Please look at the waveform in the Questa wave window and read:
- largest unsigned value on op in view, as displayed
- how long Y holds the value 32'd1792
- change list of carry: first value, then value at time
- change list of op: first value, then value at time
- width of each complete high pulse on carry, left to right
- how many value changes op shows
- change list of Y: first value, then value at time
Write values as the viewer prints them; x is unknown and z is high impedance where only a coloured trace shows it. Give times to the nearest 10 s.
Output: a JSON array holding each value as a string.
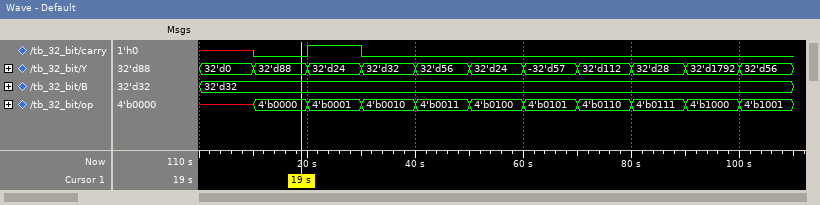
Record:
["4'b1001", "10 s", "x, 0 at 10 s, 1 at 20 s, 0 at 30 s", "x, 4'b0000 at 10 s, 4'b0001 at 20 s, 4'b0010 at 30 s, 4'b0011 at 40 s, 4'b0100 at 50 s, 4'b0101 at 60 s, 4'b0110 at 70 s, 4'b0111 at 80 s, 4'b1000 at 90 s, 4'b1001 at 100 s", "10 s", "10", "32'd0, 32'd88 at 10 s, 32'd24 at 20 s, 32'd32 at 30 s, 32'd56 at 40 s, 32'd24 at 50 s, -32'd57 at 60 s, 32'd112 at 70 s, 32'd28 at 80 s, 32'd1792 at 90 s, 32'd56 at 100 s"]
